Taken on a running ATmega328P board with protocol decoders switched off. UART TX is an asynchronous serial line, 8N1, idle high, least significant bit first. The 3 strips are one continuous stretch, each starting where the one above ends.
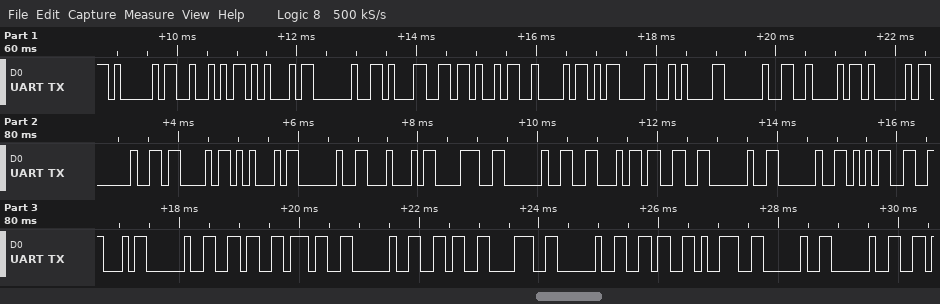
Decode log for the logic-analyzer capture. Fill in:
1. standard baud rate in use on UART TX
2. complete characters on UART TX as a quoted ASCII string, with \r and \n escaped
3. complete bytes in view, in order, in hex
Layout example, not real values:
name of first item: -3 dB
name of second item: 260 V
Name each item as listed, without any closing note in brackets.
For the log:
standard baud rate in use on UART TX: 9600 baud
complete characters on UART TX as a quoted ASCII string, with \r and \n escaped: "ARE 1KB\r\n BA CE D8 F3  5F 67 68 69  "
complete bytes in view, in order, in hex: 41 52 45 20 31 4B 42 0D 0A 20 42 41 20 43 45 20 44 38 20 46 33 20 20 35 46 20 36 37 20 36 38 20 36 39 20 20
